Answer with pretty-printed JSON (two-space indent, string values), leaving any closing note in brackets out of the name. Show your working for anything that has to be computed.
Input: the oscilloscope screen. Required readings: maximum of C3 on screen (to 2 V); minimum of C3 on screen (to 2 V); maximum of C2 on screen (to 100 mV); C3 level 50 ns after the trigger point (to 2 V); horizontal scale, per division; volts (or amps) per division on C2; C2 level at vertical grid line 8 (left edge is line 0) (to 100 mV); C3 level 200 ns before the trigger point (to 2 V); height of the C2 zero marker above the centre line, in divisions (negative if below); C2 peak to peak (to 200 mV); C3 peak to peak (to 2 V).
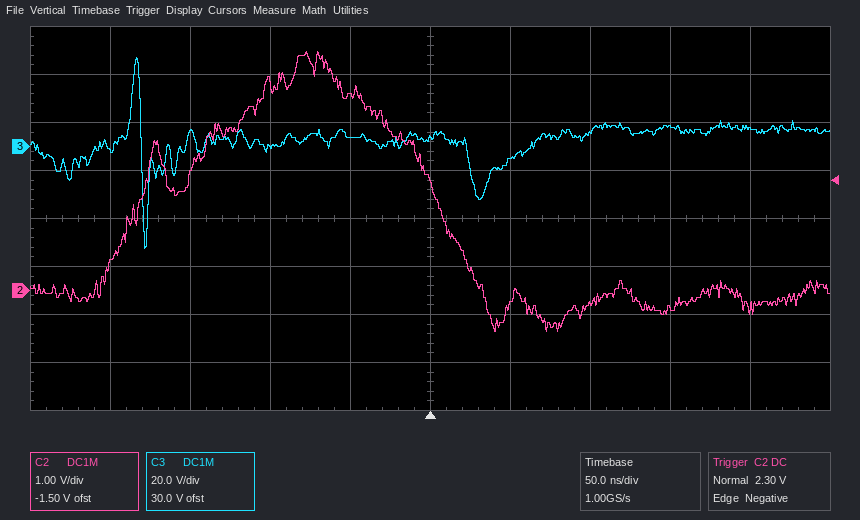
{
  "maximum of C3 on screen": "38 V",
  "minimum of C3 on screen": "-42 V",
  "maximum of C2 on screen": "5.0 V",
  "C3 level 50 ns after the trigger point": "-6 V",
  "horizontal scale, per division": "50 ns",
  "volts (or amps) per division on C2": "1 V",
  "C2 level at vertical grid line 8 (left edge is line 0)": "-400 mV",
  "C3 level 200 ns before the trigger point": "0 V",
  "height of the C2 zero marker above the centre line, in divisions": "-1.5 div",
  "C2 peak to peak": "5.8 V",
  "C3 peak to peak": "38 V − (-42 V) = 80 V"
}
